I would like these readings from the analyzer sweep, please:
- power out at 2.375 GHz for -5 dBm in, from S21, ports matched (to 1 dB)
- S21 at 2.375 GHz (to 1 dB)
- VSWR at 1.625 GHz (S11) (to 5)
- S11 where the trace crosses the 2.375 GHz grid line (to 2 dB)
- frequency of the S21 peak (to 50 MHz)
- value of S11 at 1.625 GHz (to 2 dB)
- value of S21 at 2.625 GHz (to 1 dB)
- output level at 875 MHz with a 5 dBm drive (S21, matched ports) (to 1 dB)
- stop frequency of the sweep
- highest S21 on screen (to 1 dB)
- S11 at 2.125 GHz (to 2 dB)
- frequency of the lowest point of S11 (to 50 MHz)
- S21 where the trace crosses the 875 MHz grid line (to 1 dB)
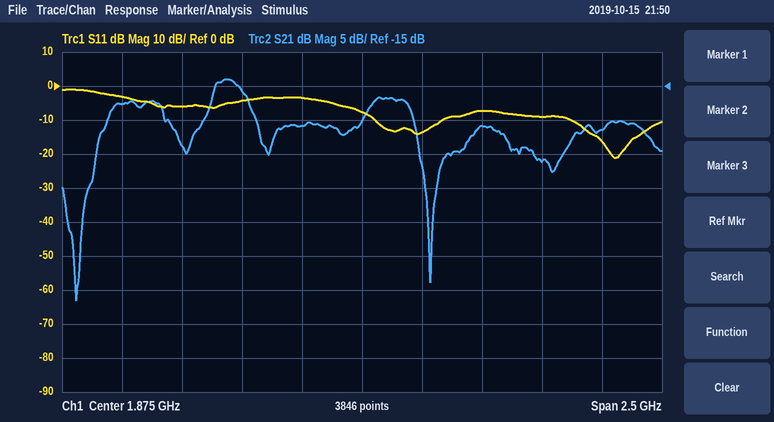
-26 dBm
-21 dB
5
-8 dB
1.30 GHz
-4 dB
-26 dB
-13 dBm
3.125 GHz
-14 dB
-14 dB
2.95 GHz
-18 dB
